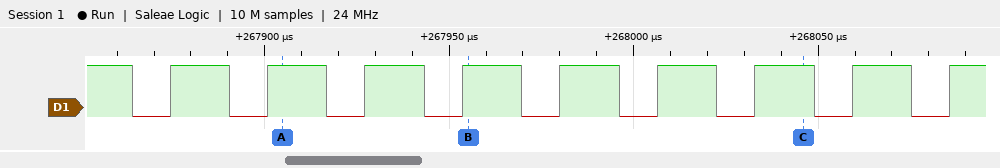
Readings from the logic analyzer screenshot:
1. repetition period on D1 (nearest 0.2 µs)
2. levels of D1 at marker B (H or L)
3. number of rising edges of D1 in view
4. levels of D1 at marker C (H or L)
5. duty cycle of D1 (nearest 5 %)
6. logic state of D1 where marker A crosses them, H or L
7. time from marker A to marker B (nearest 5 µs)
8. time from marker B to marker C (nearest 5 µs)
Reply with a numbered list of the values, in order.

1. 26.4 µs
2. D1=H
3. 9
4. D1=H
5. 60 %
6. D1=H
7. 50 µs
8. 90 µs
